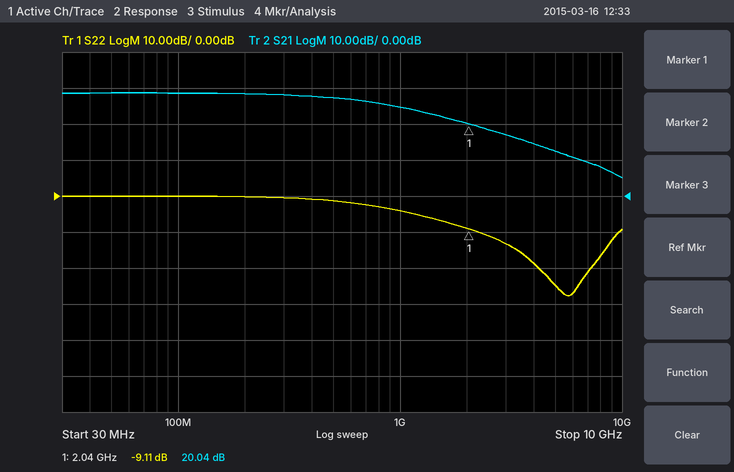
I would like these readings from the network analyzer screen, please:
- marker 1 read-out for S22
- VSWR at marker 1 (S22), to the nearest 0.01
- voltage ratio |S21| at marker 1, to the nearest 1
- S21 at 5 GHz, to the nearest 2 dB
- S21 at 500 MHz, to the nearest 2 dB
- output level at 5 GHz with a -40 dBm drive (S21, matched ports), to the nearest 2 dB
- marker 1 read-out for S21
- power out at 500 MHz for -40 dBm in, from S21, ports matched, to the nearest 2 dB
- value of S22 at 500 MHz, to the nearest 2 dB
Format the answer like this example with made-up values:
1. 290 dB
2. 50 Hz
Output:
1. -9.11 dB
2. 2.08
3. 10
4. 12 dB
5. 28 dB
6. -28 dBm
7. 20.04 dB
8. -12 dBm
9. -2 dB
